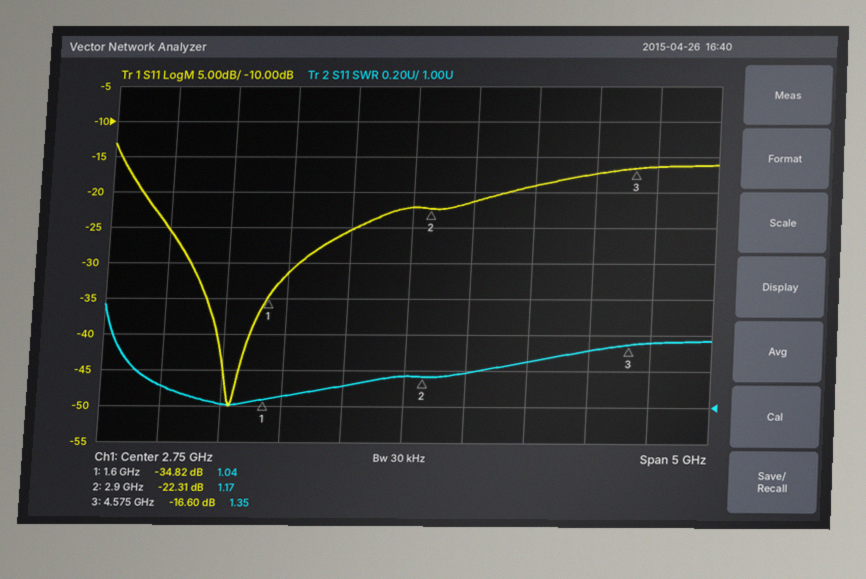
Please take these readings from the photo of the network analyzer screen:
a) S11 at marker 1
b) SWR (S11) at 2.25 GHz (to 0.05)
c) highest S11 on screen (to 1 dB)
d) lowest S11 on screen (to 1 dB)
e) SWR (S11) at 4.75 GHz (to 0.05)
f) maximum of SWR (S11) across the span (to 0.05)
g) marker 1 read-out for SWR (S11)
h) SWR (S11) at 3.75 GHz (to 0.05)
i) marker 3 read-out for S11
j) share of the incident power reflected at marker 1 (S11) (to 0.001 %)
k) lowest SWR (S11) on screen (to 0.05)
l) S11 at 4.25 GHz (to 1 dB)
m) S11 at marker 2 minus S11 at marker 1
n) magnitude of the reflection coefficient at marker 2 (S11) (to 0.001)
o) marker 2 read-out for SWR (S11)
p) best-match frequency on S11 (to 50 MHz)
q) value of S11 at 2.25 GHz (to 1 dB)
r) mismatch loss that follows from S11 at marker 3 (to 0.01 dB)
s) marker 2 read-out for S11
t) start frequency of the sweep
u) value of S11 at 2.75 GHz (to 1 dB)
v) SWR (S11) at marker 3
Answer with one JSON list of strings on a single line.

["-34.82 dB", "1.10", "-13 dB", "-50 dB", "1.35", "1.55", "1.04", "1.25", "-16.60 dB", "0.033 %", "1.00", "-17 dB", "12.51 dB", "0.077", "1.17", "1.30 GHz", "-25 dB", "0.10 dB", "-22.31 dB", "250 MHz", "-22 dB", "1.35"]
